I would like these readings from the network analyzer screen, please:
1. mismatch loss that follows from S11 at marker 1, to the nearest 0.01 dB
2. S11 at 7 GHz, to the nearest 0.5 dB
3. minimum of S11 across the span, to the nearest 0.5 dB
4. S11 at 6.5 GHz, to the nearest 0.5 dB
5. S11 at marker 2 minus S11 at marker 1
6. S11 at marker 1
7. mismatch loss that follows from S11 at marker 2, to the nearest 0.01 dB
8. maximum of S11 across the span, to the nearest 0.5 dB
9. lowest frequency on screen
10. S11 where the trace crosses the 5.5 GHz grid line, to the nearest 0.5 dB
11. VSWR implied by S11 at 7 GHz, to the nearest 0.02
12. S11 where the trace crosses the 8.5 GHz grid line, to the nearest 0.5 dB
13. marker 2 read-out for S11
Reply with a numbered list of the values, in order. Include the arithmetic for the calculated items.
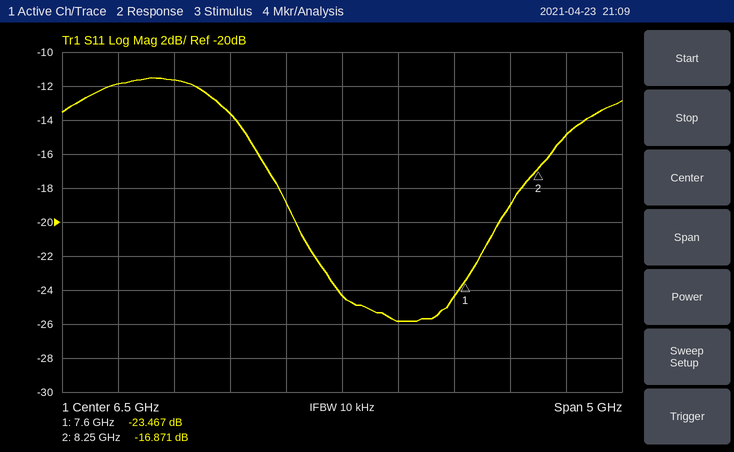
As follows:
1. −10 log10(1 − 10^(-23.467/10)) ≈ 0.02 dB
2. -26.0 dB
3. -26.0 dB
4. -24.5 dB
5. -16.871 − (-23.467) = 6.596 dB
6. -23.467 dB
7. −10 log10(1 − 10^(-16.871/10)) ≈ 0.09 dB
8. -11.5 dB
9. 4 GHz
10. -13.5 dB
11. |Γ| = 10^(-26/20) = 0.0501; VSWR = (1 + 0.0501)/(1 − 0.0501) ≈ 1.11, so 1.10 to the nearest 0.02
12. -15.0 dB
13. -16.871 dB
